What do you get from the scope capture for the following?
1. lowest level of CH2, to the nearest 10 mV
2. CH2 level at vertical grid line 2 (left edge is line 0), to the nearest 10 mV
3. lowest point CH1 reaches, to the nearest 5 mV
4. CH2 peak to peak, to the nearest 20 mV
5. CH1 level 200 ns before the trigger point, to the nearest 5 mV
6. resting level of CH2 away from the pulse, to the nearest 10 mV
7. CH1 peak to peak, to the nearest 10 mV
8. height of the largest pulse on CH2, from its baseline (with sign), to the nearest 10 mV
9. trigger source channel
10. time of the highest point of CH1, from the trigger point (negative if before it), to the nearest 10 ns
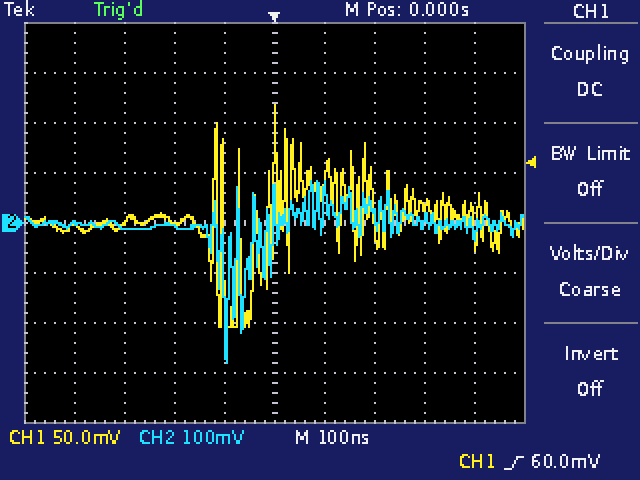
-280 mV
-10 mV
-105 mV
360 mV
0 mV
0 mV
220 mV
-280 mV
CH1
0 ns
